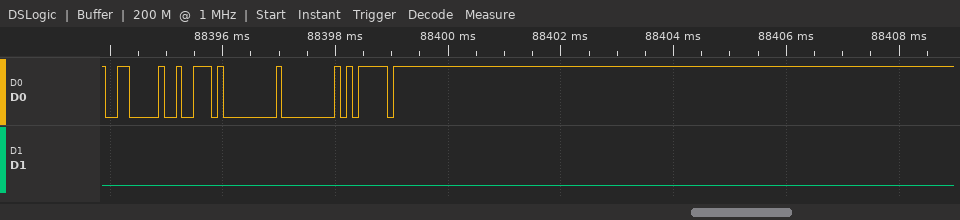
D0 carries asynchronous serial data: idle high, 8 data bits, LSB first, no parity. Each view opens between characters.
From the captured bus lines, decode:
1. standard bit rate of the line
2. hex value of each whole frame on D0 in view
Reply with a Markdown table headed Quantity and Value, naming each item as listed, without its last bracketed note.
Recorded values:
| Quantity | Value |
|---|---|
| standard bit rate of the line | 9600 baud |
| hex value of each whole frame on D0 in view | 06, 72, 00, 00, 7D |
